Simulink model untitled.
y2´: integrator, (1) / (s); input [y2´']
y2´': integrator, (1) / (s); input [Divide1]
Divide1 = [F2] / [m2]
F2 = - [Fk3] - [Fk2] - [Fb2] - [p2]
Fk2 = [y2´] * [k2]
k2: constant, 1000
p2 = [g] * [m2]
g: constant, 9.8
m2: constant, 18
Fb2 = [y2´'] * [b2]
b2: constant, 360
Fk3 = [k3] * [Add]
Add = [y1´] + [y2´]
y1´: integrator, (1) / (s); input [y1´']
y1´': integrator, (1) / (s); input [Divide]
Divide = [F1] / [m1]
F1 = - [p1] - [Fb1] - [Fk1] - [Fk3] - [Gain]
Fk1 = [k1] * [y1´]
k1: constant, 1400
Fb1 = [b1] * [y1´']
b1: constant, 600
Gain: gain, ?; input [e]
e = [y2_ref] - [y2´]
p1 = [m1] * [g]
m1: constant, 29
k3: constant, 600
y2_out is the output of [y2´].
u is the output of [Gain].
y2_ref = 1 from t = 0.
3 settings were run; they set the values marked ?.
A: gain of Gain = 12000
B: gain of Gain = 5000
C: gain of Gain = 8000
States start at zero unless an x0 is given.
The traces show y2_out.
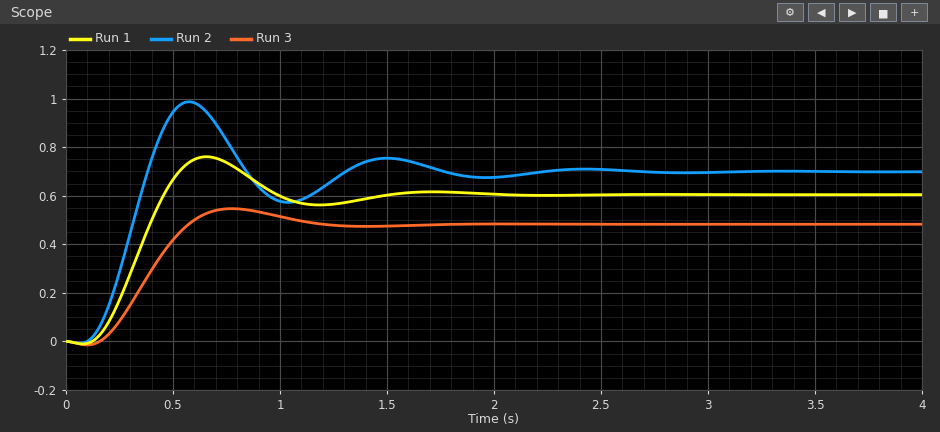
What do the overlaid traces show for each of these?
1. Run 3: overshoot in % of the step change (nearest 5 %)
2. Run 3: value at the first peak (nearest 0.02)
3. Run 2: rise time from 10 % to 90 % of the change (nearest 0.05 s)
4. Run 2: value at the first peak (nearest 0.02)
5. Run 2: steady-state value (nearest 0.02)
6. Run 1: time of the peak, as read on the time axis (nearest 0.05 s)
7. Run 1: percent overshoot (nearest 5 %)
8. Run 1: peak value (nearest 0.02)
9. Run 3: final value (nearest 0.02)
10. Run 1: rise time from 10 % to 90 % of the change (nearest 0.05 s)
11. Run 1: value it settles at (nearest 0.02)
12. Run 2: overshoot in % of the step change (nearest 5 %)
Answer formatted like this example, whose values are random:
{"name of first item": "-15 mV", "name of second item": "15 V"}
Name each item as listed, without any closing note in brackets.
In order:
{"Run 3: overshoot in % of the step change": "15 %", "Run 3: value at the first peak": "0.54", "Run 2: rise time from 10 % to 90 % of the change": "0.20 s", "Run 2: value at the first peak": "0.98", "Run 2: steady-state value": "0.70", "Run 1: time of the peak, as read on the time axis": "0.65 s", "Run 1: percent overshoot": "25 %", "Run 1: peak value": "0.76", "Run 3: final value": "0.48", "Run 1: rise time from 10 % to 90 % of the change": "0.25 s", "Run 1: value it settles at": "0.60", "Run 2: overshoot in % of the step change": "40 %"}
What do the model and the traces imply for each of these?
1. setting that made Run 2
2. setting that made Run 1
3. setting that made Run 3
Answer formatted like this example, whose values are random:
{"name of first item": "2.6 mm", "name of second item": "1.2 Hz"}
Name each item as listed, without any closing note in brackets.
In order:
{"setting that made Run 2": "A", "setting that made Run 1": "C", "setting that made Run 3": "B"}
